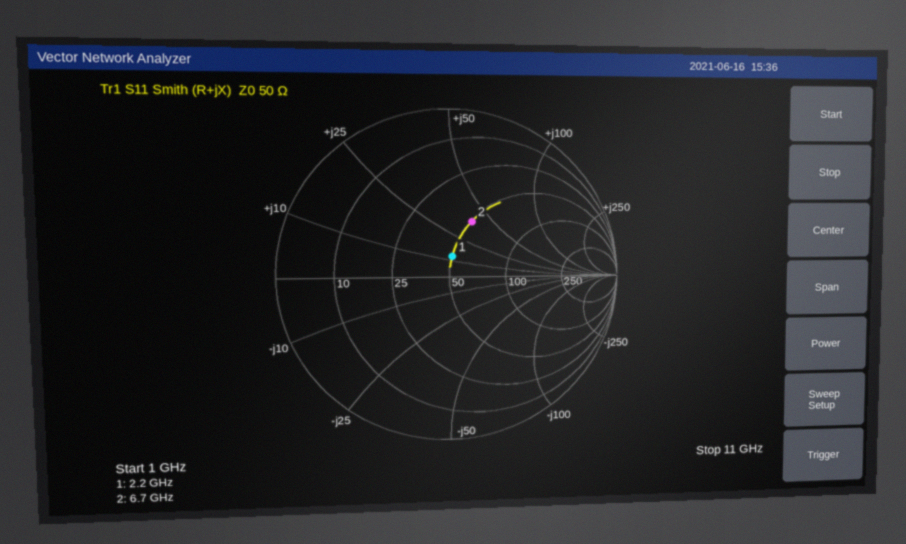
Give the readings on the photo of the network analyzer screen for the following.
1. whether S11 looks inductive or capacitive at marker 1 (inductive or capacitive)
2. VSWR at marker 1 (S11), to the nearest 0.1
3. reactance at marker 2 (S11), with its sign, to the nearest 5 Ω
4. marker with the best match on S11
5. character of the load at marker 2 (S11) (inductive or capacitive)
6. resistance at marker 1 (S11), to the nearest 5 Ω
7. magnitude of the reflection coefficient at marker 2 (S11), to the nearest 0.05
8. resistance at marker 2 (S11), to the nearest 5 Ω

inductive
1.3
+40 Ω
marker 1
inductive
50 Ω
0.35
50 Ω
